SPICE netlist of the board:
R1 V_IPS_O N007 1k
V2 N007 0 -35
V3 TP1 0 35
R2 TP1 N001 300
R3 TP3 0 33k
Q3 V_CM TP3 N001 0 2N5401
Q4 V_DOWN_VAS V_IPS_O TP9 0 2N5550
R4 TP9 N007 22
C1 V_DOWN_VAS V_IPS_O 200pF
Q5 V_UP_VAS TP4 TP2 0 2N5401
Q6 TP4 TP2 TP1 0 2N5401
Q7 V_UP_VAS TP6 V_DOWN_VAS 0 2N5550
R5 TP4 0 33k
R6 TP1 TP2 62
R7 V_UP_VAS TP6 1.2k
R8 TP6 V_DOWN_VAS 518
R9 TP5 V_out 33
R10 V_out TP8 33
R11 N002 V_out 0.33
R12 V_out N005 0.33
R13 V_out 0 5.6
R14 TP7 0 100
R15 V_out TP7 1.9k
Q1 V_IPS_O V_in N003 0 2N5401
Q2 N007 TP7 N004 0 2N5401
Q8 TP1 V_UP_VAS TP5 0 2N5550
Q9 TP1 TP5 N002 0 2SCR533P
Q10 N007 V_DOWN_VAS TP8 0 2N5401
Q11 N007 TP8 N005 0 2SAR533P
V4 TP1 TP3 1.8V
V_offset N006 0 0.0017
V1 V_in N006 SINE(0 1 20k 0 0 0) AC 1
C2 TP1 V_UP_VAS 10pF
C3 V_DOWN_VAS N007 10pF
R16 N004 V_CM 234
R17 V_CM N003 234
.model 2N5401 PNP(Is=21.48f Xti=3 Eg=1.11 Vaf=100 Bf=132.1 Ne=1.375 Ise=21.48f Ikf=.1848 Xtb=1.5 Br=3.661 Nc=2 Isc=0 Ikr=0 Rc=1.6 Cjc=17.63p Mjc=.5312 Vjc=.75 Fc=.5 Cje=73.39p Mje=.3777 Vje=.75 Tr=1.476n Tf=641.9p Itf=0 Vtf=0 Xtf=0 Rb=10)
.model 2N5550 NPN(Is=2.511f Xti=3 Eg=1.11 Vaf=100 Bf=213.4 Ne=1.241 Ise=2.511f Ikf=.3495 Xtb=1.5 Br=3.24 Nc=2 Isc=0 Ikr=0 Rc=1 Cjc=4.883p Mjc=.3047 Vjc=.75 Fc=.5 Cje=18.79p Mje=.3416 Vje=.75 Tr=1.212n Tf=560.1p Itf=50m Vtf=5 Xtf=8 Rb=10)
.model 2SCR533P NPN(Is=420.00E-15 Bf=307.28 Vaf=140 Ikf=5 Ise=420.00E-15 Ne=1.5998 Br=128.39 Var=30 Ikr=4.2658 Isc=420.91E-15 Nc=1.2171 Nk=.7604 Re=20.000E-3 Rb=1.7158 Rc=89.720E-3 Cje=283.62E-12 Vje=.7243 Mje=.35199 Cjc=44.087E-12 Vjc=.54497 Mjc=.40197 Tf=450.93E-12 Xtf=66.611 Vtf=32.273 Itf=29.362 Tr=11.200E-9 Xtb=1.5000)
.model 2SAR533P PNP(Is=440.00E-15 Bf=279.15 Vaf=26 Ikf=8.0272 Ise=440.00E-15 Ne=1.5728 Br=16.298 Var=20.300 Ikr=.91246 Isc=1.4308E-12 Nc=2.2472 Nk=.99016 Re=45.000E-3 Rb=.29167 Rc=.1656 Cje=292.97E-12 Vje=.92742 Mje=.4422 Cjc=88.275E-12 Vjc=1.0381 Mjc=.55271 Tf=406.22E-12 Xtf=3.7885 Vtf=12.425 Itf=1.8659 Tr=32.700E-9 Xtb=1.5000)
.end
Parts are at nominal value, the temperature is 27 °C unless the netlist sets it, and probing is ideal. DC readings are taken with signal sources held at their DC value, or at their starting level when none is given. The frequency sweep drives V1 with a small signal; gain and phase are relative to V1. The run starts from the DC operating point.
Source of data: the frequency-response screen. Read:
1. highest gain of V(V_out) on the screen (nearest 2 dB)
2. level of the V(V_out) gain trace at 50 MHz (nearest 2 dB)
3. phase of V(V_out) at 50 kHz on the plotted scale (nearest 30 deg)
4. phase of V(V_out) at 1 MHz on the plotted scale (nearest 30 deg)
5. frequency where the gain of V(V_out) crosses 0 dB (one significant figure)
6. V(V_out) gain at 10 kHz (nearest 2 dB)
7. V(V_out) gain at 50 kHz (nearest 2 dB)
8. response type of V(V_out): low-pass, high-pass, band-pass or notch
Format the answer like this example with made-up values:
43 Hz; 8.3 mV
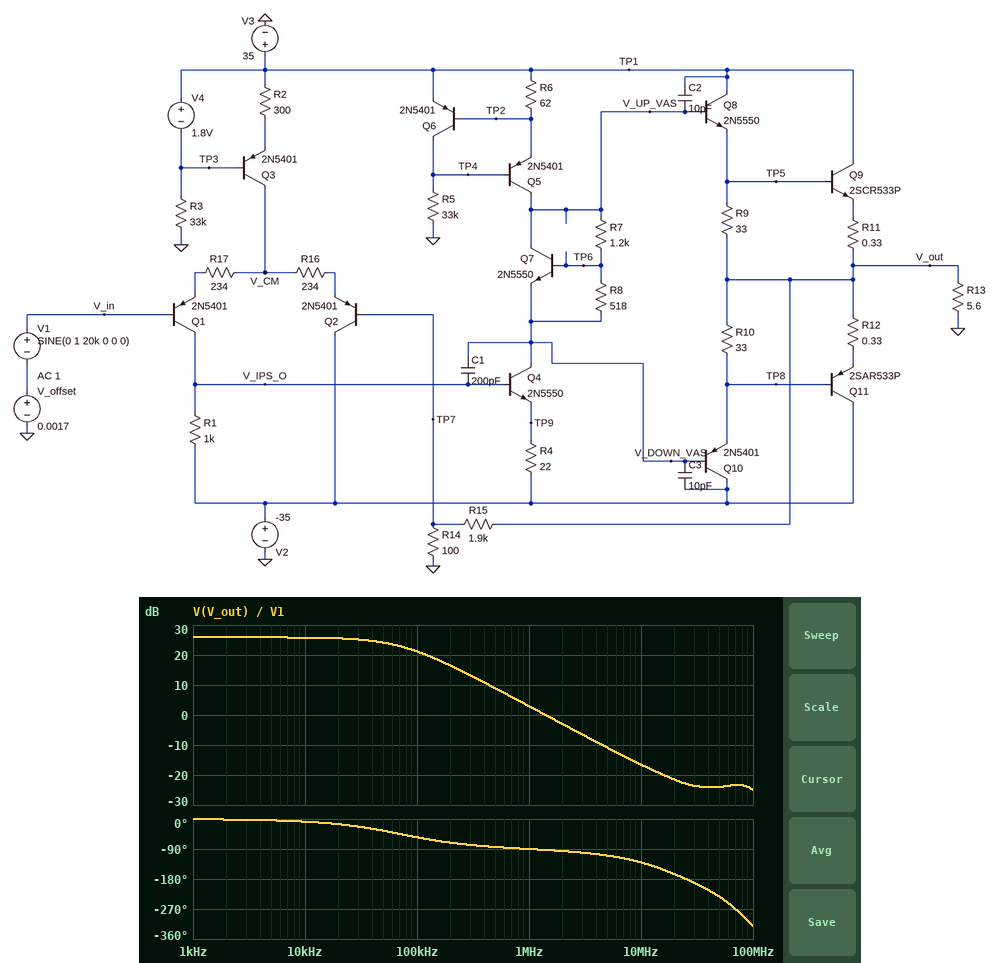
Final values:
26 dB; -24 dB; -30 deg; -90 deg; 1 MHz; 26 dB; 24 dB; low-pass
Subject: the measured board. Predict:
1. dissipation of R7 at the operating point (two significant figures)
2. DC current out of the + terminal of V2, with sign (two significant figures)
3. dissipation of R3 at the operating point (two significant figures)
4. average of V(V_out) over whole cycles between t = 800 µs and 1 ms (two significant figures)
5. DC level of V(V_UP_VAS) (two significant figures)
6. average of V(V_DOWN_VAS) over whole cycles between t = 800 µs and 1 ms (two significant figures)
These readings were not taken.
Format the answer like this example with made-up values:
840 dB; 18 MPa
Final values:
2.8 mW; -1.5 A; 33 mW; -8.1 V; -7.6 V; -10 V
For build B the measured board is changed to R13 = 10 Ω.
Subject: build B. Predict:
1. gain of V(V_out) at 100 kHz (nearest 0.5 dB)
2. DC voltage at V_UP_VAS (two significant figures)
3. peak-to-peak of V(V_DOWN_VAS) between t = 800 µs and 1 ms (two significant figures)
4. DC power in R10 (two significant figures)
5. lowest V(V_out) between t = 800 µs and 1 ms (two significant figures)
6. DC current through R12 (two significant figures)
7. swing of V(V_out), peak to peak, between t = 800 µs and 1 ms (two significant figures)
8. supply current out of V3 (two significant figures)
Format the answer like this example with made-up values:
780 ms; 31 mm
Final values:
21.5 dB; -7.4 V; 40 V; 31 mW; -27 V; 800 mA; 38 V; 19 mA
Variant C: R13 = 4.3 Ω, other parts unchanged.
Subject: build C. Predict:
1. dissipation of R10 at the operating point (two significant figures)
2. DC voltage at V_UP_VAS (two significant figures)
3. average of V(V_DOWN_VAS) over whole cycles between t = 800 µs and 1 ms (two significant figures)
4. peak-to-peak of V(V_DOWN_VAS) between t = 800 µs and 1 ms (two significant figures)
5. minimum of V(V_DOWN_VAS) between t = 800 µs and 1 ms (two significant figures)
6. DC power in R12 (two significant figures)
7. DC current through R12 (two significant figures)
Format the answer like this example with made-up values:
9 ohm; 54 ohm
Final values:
63 mW; -7.8 V; -9.7 V; 38 V; -28 V; 1.1 W; 1.9 A
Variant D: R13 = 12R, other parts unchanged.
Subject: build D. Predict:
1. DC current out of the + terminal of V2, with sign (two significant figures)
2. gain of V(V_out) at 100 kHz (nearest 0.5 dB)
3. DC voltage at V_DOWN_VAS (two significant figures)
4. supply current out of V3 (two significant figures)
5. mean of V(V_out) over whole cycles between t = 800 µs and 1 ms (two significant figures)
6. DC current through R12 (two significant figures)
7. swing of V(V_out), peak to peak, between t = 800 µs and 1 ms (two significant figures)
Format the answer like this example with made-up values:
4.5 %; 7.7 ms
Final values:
-710 mA; 21.5 dB; -9.9 V; 21 mA; -8.3 V; 670 mA; 38 V
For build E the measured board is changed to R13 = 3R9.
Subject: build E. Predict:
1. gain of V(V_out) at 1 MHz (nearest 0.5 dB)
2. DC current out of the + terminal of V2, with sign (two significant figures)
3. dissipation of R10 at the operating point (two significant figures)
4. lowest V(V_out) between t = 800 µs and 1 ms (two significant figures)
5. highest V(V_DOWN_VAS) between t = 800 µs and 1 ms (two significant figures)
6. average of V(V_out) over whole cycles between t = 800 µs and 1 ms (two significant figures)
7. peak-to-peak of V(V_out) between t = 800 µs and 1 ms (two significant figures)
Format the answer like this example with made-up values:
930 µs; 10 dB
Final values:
2.5 dB; -2.1 A; 70 mW; -23 V; 11 V; -7.4 V; 33 V
